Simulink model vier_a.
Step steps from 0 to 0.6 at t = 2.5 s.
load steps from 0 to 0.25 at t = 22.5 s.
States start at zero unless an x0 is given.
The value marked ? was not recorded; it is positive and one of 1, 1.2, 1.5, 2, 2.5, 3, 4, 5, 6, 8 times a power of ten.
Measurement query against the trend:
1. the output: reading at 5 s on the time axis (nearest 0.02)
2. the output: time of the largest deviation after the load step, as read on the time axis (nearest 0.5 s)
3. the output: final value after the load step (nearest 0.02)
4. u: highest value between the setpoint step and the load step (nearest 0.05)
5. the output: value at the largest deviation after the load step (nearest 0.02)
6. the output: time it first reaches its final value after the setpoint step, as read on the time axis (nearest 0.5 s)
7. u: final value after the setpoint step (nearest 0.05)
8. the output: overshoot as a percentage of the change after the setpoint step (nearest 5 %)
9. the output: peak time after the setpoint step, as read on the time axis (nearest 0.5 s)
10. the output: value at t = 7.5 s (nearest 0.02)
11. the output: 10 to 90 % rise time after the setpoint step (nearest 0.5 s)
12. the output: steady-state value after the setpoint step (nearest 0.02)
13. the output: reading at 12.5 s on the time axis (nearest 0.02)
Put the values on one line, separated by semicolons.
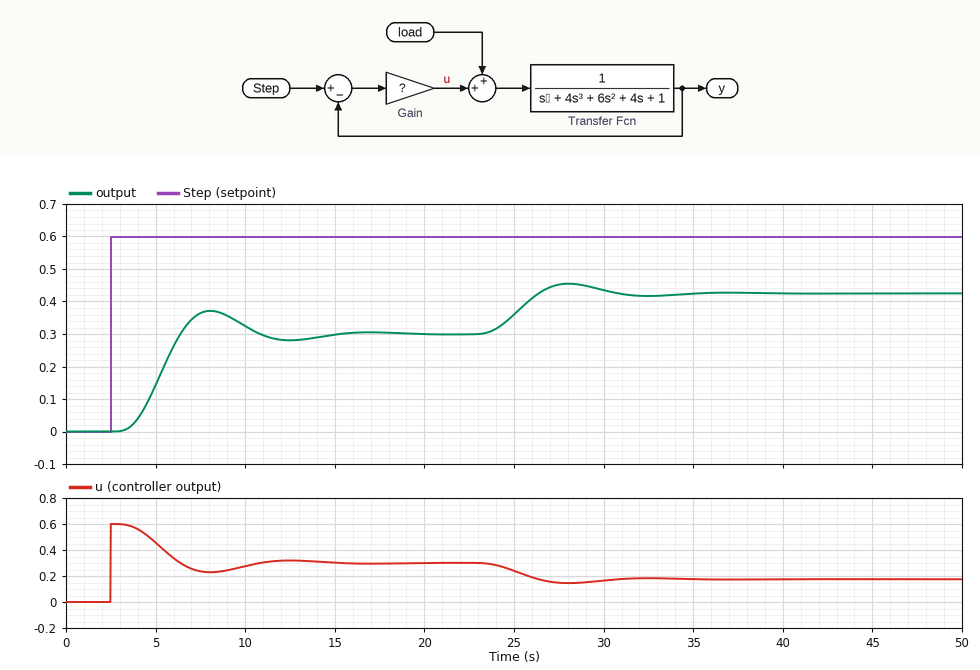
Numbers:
0.14; 28.0 s; 0.42; 0.60; 0.46; 6.5 s; 0.30; 25 %; 8.0 s; 0.36; 2.0 s; 0.30; 0.28
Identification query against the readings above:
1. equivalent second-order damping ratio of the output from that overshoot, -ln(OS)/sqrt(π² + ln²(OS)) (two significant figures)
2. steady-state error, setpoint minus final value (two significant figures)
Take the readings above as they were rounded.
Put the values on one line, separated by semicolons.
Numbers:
0.40; 0.30
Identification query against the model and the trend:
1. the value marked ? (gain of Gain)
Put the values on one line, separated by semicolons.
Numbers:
1
